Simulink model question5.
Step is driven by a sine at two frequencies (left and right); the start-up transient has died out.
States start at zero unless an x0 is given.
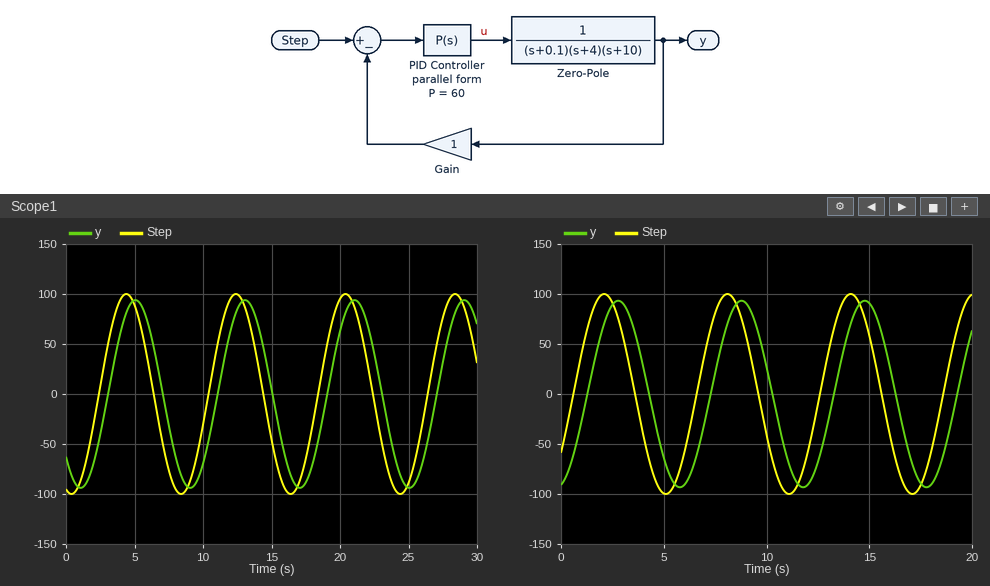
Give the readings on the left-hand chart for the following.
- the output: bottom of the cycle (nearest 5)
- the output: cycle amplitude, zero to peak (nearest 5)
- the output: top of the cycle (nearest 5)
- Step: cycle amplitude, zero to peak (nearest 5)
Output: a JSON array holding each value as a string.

["-95", "95", "95", "100"]
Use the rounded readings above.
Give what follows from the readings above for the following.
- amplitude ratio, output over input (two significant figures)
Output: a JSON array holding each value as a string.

["0.95"]
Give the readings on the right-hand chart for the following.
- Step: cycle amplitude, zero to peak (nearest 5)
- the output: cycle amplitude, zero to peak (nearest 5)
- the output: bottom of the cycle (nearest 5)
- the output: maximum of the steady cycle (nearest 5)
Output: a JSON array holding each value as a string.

["100", "95", "-95", "95"]
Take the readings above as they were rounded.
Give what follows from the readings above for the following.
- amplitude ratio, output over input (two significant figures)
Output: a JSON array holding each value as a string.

["0.95"]
